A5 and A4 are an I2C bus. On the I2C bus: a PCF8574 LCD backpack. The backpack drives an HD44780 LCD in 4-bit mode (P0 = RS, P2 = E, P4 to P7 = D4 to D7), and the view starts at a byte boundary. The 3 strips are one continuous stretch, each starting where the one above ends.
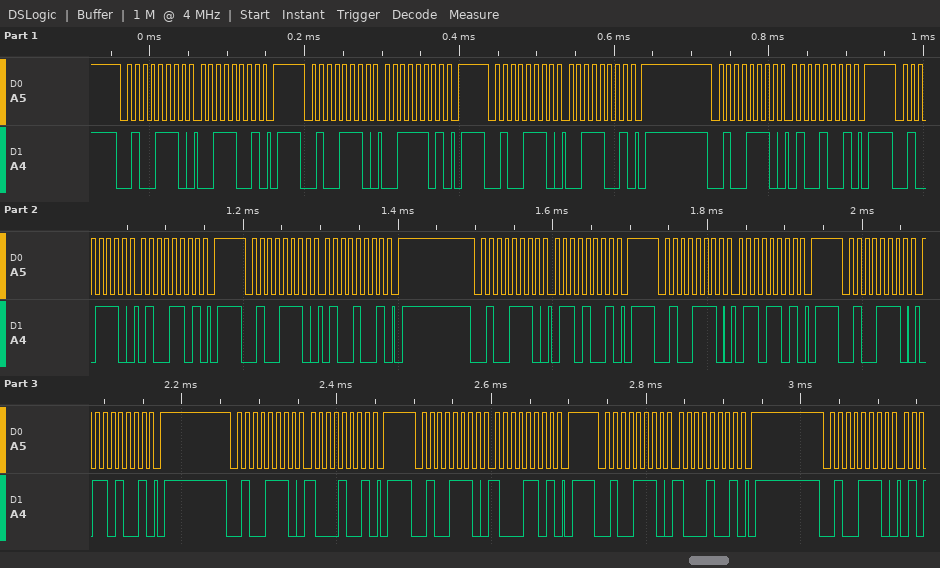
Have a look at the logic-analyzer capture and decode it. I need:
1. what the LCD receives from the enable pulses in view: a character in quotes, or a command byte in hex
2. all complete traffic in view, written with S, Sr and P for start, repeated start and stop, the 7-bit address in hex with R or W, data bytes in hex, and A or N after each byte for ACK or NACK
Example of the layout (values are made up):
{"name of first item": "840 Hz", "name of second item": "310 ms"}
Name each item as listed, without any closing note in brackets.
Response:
{"what the LCD receives from the enable pulses in view: a character in quotes, or a command byte in hex": "'4' 'h'", "all complete traffic in view, written with S, Sr and P for start, repeated start and stop, the 7-bit address in hex with R or W, data bytes in hex, and A or N after each byte for ACK or NACK": "S 27W A 39 A P S 27W A 3D A P S 27W A 39 A P S 27W A 49 A P S 27W A 4D A P S 27W A 49 A P S 27W A 69 A P S 27W A 6D A P S 27W A 69 A P S 27W A 89 A P S 27W A 8D A P S 27W A 89 A P S 27W A"}
